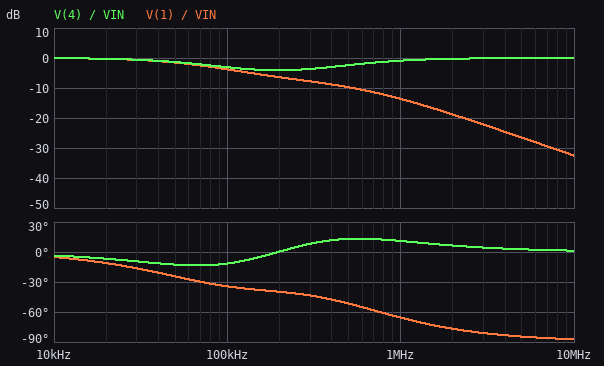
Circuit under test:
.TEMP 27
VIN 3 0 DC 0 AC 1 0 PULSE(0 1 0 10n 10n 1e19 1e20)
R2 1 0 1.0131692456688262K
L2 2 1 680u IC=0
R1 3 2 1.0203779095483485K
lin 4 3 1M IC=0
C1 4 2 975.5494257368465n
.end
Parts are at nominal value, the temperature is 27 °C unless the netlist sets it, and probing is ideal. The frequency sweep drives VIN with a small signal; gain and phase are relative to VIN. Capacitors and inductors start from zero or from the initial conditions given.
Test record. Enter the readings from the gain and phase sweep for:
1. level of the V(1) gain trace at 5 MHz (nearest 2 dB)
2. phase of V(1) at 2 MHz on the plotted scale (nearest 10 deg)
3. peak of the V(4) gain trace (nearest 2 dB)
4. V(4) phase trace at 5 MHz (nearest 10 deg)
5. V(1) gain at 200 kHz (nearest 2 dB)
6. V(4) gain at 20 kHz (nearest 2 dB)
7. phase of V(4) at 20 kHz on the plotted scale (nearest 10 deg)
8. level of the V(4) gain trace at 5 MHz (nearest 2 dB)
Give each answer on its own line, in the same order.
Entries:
-26 dB
-80 deg
0 dB
0 deg
-6 dB
0 dB
-10 deg
0 dB
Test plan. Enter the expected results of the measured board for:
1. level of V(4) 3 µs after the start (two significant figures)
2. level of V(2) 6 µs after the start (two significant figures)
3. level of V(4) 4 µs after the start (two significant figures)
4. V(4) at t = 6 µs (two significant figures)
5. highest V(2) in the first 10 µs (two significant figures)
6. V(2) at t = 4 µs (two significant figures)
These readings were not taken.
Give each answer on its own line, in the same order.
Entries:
870 mV
960 mV
910 mV
960 mV
990 mV
910 mV
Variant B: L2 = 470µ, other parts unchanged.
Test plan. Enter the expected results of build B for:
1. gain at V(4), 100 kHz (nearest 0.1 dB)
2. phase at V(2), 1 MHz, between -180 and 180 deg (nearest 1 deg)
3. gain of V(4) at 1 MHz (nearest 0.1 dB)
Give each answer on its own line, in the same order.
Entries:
-3.0 dB
14 deg
-1.5 dB
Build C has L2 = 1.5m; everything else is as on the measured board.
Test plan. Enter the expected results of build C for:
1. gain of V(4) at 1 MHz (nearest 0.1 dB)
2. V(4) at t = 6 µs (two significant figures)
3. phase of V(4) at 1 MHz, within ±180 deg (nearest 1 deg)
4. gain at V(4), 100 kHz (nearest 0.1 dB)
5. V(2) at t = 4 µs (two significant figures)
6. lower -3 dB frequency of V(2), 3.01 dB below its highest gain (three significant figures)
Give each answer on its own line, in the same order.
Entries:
-0.3 dB
950 mV
6 deg
-2.8 dB
900 mV
227 Hz
